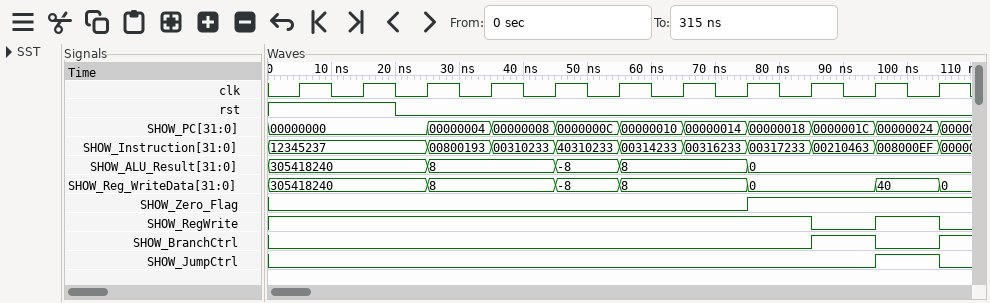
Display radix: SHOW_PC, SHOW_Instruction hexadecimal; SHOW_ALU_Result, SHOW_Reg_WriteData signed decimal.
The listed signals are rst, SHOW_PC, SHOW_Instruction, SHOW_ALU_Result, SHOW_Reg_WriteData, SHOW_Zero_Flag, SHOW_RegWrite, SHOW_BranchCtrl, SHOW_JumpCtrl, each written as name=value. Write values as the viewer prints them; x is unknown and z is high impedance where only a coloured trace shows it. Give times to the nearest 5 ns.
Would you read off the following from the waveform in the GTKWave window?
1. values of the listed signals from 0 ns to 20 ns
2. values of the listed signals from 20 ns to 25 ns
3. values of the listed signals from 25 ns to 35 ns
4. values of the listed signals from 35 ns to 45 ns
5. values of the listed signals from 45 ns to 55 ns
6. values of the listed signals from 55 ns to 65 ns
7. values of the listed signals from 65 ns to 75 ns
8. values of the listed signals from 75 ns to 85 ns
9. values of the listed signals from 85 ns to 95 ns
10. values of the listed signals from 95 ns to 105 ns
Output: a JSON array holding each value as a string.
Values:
["rst=1, SHOW_PC=00000000, SHOW_Instruction=12345237, SHOW_ALU_Result=305418240, SHOW_Reg_WriteData=305418240, SHOW_Zero_Flag=0, SHOW_RegWrite=1, SHOW_BranchCtrl=0, SHOW_JumpCtrl=0", "rst=0, SHOW_PC=00000000, SHOW_Instruction=12345237, SHOW_ALU_Result=305418240, SHOW_Reg_WriteData=305418240, SHOW_Zero_Flag=0, SHOW_RegWrite=1, SHOW_BranchCtrl=0, SHOW_JumpCtrl=0", "rst=0, SHOW_PC=00000004, SHOW_Instruction=00800193, SHOW_ALU_Result=8, SHOW_Reg_WriteData=8, SHOW_Zero_Flag=0, SHOW_RegWrite=1, SHOW_BranchCtrl=0, SHOW_JumpCtrl=0", "rst=0, SHOW_PC=00000008, SHOW_Instruction=00310233, SHOW_ALU_Result=8, SHOW_Reg_WriteData=8, SHOW_Zero_Flag=0, SHOW_RegWrite=1, SHOW_BranchCtrl=0, SHOW_JumpCtrl=0", "rst=0, SHOW_PC=0000000C, SHOW_Instruction=40310233, SHOW_ALU_Result=-8, SHOW_Reg_WriteData=-8, SHOW_Zero_Flag=0, SHOW_RegWrite=1, SHOW_BranchCtrl=0, SHOW_JumpCtrl=0", "rst=0, SHOW_PC=00000010, SHOW_Instruction=00314233, SHOW_ALU_Result=8, SHOW_Reg_WriteData=8, SHOW_Zero_Flag=0, SHOW_RegWrite=1, SHOW_BranchCtrl=0, SHOW_JumpCtrl=0", "rst=0, SHOW_PC=00000014, SHOW_Instruction=00316233, SHOW_ALU_Result=8, SHOW_Reg_WriteData=8, SHOW_Zero_Flag=0, SHOW_RegWrite=1, SHOW_BranchCtrl=0, SHOW_JumpCtrl=0", "rst=0, SHOW_PC=00000018, SHOW_Instruction=00317233, SHOW_ALU_Result=0, SHOW_Reg_WriteData=0, SHOW_Zero_Flag=1, SHOW_RegWrite=1, SHOW_BranchCtrl=0, SHOW_JumpCtrl=0", "rst=0, SHOW_PC=0000001C, SHOW_Instruction=00210463, SHOW_ALU_Result=0, SHOW_Reg_WriteData=0, SHOW_Zero_Flag=1, SHOW_RegWrite=0, SHOW_BranchCtrl=1, SHOW_JumpCtrl=0", "rst=0, SHOW_PC=00000024, SHOW_Instruction=008000EF, SHOW_ALU_Result=0, SHOW_Reg_WriteData=40, SHOW_Zero_Flag=1, SHOW_RegWrite=1, SHOW_BranchCtrl=0, SHOW_JumpCtrl=1"]
